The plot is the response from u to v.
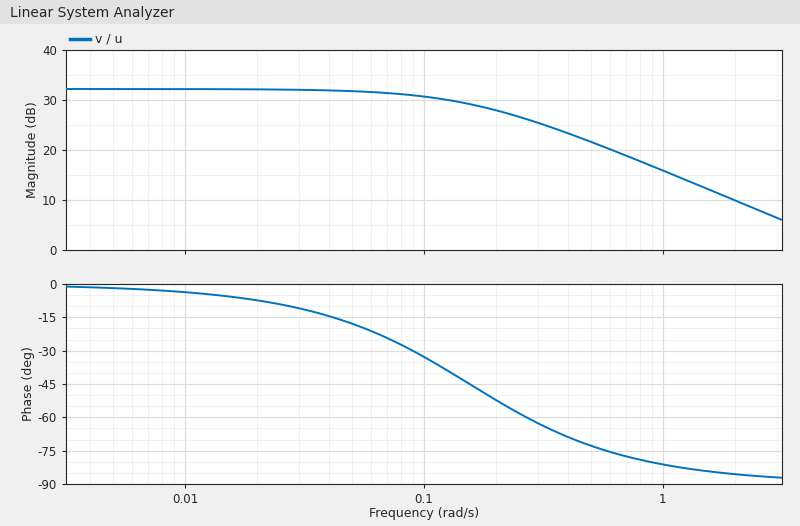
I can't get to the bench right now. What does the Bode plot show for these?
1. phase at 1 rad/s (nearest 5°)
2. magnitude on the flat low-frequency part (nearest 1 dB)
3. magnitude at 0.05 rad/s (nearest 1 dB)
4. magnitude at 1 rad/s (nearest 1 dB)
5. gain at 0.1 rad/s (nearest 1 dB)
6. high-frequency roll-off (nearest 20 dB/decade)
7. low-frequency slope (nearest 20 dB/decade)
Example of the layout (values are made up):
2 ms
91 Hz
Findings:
-80°
32 dB
32 dB
16 dB
31 dB
-20 dB/decade
0 dB/decade
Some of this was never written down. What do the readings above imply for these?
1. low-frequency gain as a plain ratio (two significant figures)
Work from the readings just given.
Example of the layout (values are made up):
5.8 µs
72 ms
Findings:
40
